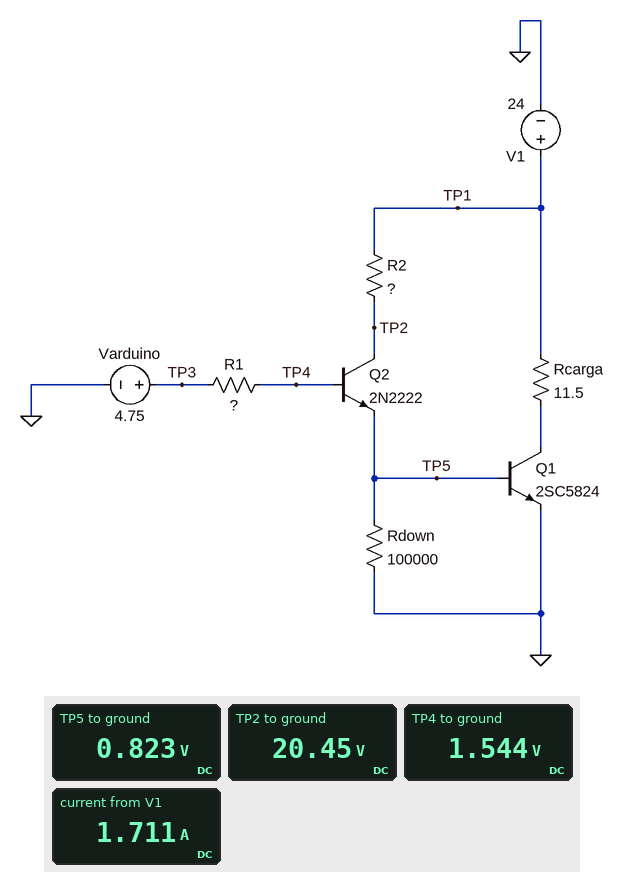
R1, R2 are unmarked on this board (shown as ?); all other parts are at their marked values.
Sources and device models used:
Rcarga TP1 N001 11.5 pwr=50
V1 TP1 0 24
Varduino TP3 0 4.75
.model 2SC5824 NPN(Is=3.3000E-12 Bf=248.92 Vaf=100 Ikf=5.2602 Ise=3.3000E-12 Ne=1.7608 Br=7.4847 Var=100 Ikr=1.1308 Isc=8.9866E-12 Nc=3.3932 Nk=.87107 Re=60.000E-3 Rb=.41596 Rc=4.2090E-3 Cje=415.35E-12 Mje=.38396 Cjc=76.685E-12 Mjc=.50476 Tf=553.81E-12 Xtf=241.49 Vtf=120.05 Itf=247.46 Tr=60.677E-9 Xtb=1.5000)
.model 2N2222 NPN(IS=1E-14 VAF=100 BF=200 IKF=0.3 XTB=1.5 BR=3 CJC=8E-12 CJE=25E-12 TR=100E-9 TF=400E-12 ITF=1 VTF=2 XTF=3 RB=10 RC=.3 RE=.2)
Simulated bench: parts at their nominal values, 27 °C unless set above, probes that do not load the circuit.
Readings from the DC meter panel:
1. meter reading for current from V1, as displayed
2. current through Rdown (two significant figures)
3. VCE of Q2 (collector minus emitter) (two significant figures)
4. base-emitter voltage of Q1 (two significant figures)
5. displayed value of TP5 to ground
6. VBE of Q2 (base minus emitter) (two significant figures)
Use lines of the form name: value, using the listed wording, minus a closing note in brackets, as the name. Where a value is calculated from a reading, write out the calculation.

meter reading for current from V1, as displayed: 1.711 A
current through Rdown: (823 mV) / 100 kΩ = 8.2 µA
VCE of Q2 (collector minus emitter): 20.45 V - 823 mV = 20 V
base-emitter voltage of Q1: 823 mV = 820 mV
displayed value of TP5 to ground: 0.823 V
VBE of Q2 (base minus emitter): 1.544 V - 823 mV = 720 mV
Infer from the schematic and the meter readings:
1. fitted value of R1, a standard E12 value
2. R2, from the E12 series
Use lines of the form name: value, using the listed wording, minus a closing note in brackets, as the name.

fitted value of R1, a standard E12 value: 56 kΩ
R2, from the E12 series: 270 Ω
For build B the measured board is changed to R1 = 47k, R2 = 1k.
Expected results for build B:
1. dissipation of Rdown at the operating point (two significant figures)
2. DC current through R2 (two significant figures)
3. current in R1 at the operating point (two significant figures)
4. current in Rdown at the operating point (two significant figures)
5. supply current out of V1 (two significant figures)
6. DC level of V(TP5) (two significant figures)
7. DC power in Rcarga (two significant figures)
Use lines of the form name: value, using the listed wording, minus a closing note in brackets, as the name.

dissipation of Rdown at the operating point: 6.9 µW
DC current through R2: 14 mA
current in R1 at the operating point: 68 µA
current in Rdown at the operating point: 8.3 µA
supply current out of V1: 1.8 A
DC level of V(TP5): 830 mV
DC power in Rcarga: 35 W
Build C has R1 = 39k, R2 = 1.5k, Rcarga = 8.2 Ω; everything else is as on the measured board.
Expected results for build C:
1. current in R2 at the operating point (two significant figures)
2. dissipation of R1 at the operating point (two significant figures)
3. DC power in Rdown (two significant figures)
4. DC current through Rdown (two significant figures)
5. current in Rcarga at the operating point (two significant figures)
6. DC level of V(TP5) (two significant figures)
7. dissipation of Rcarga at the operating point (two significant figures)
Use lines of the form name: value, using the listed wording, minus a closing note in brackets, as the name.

current in R2 at the operating point: 15 mA
dissipation of R1 at the operating point: 260 µW
DC power in Rdown: 7.1 µW
DC current through Rdown: 8.4 µA
current in Rcarga at the operating point: 1.9 A
DC level of V(TP5): 840 mV
dissipation of Rcarga at the operating point: 30 W
